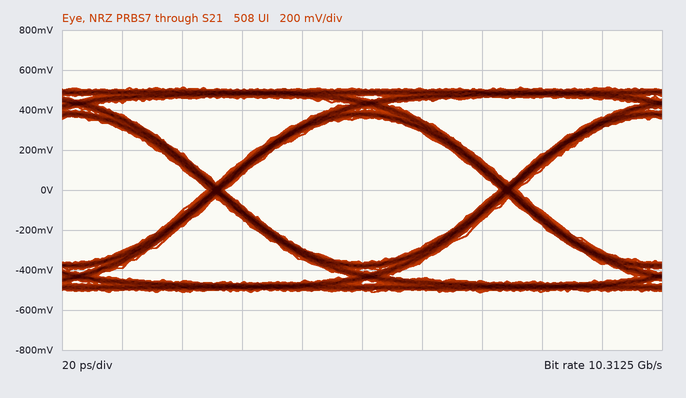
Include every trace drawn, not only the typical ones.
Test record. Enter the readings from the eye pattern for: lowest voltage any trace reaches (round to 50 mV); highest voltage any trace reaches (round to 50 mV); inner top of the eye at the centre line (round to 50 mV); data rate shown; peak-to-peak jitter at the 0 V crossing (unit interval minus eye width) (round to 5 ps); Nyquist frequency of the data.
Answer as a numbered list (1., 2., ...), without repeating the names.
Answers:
1. -500 mV
2. 500 mV
3. 350 mV
4. 10.3125 Gb/s
5. 5 ps
6. 5.15625 GHz
